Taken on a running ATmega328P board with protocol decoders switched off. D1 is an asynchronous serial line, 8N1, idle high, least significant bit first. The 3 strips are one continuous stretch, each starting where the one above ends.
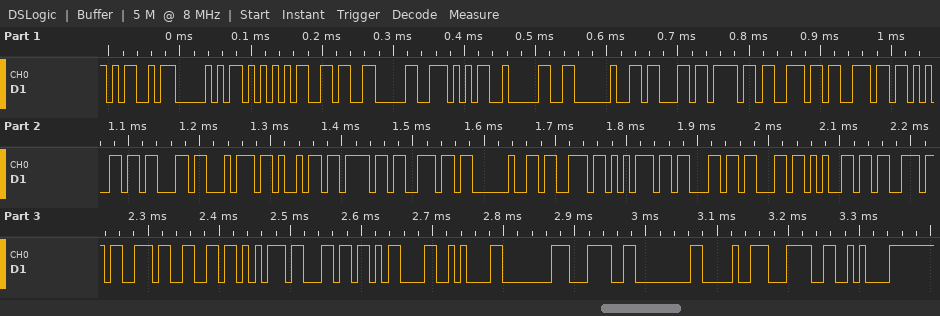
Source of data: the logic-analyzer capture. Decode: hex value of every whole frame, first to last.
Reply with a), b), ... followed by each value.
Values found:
a) 4D 50 55 36 30 35 30 20 63 6F 6E 6E 65 63 74 69 6F 6E 20 73 75 63 63 65 73 73 66 75 6C 0D 0A 80 3C 00 90 3C 0A
